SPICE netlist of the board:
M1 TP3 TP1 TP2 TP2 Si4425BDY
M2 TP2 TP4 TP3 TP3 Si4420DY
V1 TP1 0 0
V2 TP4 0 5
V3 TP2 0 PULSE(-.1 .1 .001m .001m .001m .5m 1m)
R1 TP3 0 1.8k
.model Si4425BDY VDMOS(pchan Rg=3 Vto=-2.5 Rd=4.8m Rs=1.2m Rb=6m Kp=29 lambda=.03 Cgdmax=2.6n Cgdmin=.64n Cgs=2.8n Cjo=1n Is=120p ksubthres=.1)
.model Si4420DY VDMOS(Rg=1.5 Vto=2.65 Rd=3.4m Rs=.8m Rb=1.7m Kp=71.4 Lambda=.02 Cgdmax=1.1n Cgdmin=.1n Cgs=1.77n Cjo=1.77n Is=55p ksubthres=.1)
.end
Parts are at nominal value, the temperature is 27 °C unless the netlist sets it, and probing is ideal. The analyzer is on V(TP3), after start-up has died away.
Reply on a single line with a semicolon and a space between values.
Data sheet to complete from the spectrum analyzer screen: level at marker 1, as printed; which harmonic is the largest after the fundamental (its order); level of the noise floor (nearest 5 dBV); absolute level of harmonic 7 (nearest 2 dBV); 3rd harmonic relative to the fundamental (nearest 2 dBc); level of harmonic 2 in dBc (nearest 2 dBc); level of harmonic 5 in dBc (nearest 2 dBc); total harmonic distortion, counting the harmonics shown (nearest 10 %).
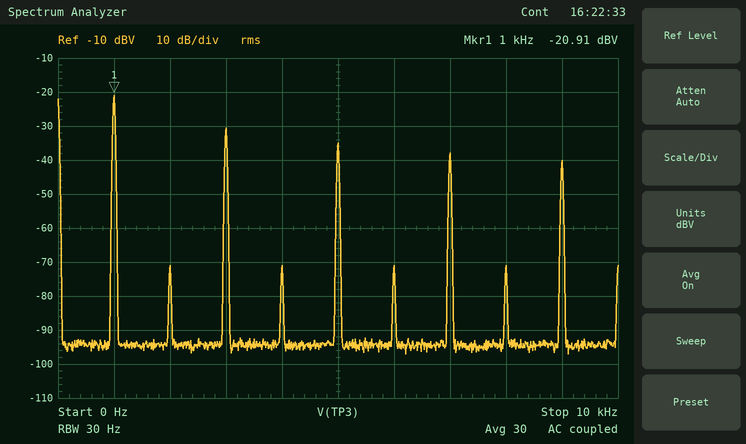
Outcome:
-20.91 dBV; 3; -95 dBV; -38 dBV; -10 dBc; -50 dBc; -14 dBc; 40 %
